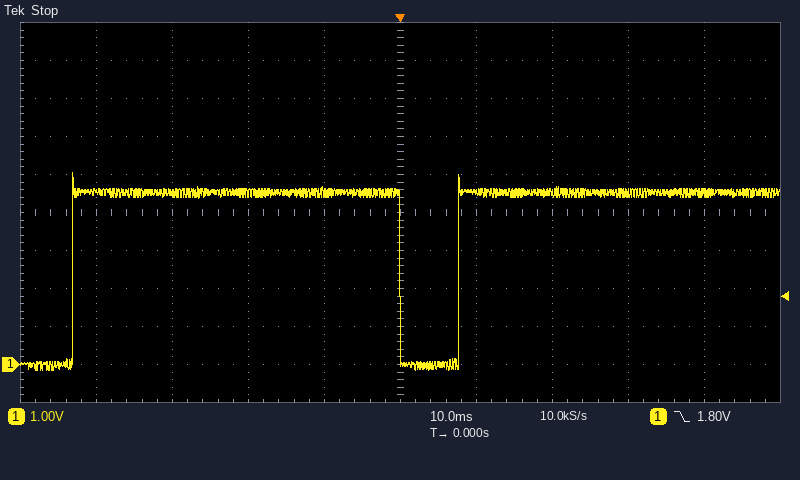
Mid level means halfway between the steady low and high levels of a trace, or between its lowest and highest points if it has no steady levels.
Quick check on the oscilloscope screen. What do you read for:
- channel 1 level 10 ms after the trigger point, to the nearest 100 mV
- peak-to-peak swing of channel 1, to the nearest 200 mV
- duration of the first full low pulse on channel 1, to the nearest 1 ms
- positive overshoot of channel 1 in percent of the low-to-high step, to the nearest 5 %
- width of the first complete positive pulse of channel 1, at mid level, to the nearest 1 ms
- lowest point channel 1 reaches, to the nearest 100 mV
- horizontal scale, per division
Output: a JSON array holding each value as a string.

["4.5 V", "5.2 V", "8 ms", "10 %", "43 ms", "-200 mV", "10 ms"]
